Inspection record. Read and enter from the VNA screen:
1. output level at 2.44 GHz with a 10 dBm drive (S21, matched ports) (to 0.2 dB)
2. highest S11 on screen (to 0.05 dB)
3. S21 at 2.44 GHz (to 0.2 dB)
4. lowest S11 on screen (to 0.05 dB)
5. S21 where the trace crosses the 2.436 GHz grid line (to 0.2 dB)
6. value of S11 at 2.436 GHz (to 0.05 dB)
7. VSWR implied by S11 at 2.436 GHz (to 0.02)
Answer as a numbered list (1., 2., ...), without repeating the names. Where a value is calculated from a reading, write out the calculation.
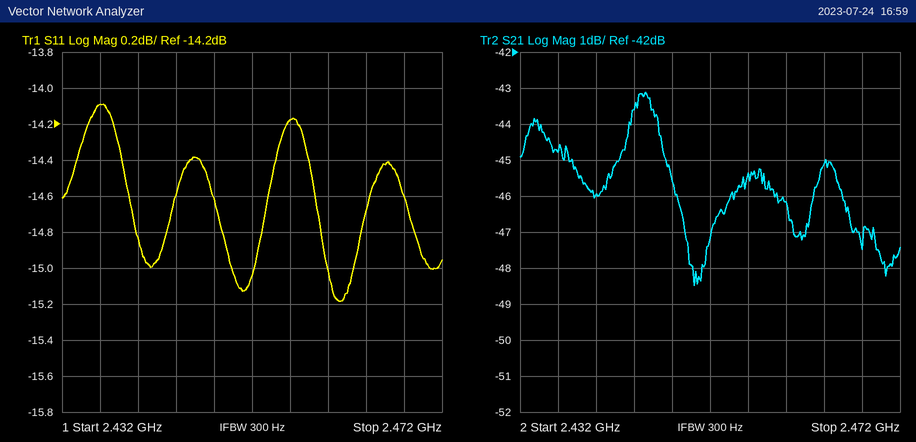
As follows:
1. 10 dBm + (-46.0 dB) = -36.0 dBm
2. -14.10 dB
3. -46.0 dB
4. -15.20 dB
5. -44.8 dB
6. -14.10 dB
7. |Γ| = 10^(-14.1/20) = 0.1972; VSWR = (1 + 0.1972)/(1 − 0.1972) ≈ 1.49, so 1.50 to the nearest 0.02
